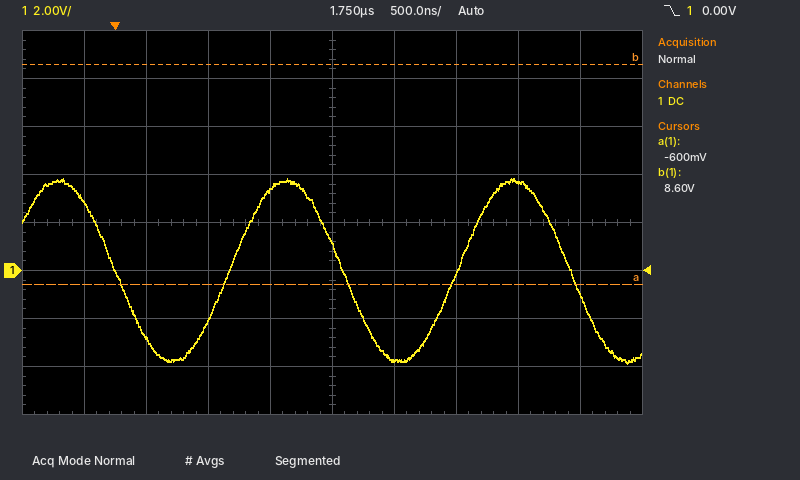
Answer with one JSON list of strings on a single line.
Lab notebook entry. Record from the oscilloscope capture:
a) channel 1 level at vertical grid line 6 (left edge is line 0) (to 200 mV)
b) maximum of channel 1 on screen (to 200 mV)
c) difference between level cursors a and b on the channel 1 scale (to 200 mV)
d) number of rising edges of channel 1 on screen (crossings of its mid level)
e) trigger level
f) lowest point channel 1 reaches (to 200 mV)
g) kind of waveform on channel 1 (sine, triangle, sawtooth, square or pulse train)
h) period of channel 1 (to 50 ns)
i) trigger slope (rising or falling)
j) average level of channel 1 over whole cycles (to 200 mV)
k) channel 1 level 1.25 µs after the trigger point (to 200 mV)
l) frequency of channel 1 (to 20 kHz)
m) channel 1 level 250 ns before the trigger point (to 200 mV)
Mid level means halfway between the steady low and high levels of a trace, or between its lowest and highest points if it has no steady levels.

["-3.8 V", "3.8 V", "9.2 V", "2", "0.00 V", "-3.8 V", "sine", "1.85 µs", "falling", "0.0 V", "3.4 V", "540 kHz", "2.8 V"]
